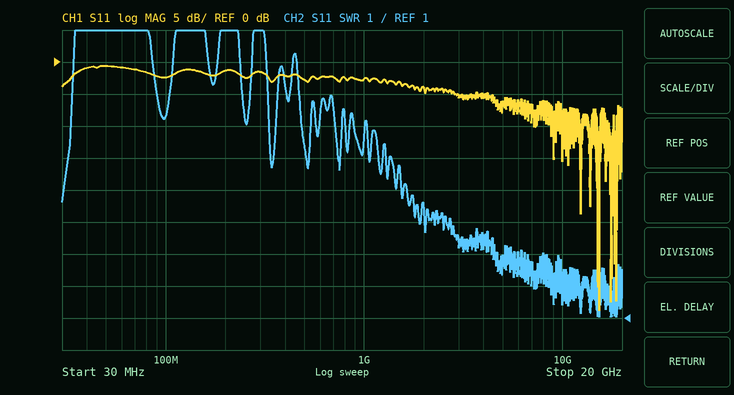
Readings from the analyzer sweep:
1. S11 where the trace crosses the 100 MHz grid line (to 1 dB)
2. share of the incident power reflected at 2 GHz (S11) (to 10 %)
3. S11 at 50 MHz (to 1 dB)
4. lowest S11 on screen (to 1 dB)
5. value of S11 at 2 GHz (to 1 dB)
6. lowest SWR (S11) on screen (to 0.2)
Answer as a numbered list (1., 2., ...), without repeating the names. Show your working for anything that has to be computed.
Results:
1. -2 dB
2. 10^(-4/10) ≈ 40 %
3. -1 dB
4. -39 dB
5. -4 dB
6. 1.0
